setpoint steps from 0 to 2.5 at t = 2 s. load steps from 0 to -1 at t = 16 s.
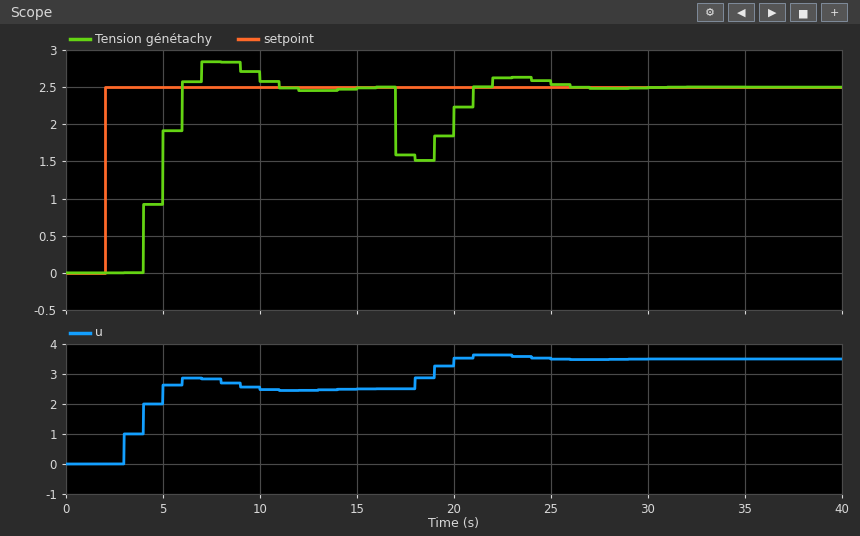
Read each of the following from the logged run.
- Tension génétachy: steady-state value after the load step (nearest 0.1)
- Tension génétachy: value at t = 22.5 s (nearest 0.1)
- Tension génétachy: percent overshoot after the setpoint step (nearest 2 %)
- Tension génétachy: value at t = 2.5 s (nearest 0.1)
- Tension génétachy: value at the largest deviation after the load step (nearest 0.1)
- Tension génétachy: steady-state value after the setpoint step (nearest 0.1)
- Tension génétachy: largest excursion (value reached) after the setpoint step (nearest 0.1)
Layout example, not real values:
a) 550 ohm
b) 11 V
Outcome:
a) 2.5
b) 2.6
c) 14 %
d) 0.0
e) 1.5
f) 2.5
g) 2.8
